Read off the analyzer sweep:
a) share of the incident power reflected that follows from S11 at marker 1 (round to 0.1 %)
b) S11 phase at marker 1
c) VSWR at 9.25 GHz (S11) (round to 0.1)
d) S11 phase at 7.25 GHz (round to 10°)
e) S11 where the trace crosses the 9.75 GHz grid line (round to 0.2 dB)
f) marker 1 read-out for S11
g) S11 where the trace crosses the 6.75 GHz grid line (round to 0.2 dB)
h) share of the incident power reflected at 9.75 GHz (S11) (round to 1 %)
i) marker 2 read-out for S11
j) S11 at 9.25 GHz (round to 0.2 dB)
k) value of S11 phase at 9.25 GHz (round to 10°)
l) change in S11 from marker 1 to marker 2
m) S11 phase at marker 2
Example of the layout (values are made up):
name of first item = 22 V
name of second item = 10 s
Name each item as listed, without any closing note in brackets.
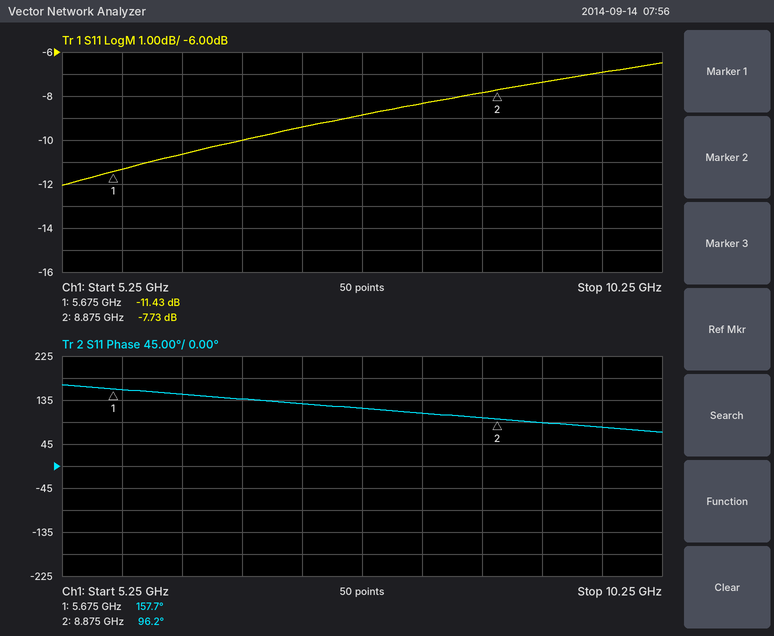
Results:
share of the incident power reflected that follows from S11 at marker 1 = 7.2 %
S11 phase at marker 1 = 157.7°
VSWR at 9.25 GHz (S11) = 2.5
S11 phase at 7.25 GHz = 130°
S11 where the trace crosses the 9.75 GHz grid line = -7.0 dB
marker 1 read-out for S11 = -11.43 dB
S11 where the trace crosses the 6.75 GHz grid line = -10.0 dB
share of the incident power reflected at 9.75 GHz (S11) = 20 %
marker 2 read-out for S11 = -7.73 dB
S11 at 9.25 GHz = -7.4 dB
value of S11 phase at 9.25 GHz = 90°
change in S11 from marker 1 to marker 2 = 3.70 dB
S11 phase at marker 2 = 96.2°
